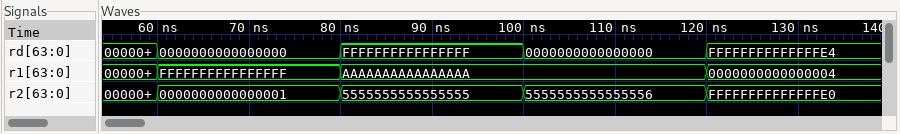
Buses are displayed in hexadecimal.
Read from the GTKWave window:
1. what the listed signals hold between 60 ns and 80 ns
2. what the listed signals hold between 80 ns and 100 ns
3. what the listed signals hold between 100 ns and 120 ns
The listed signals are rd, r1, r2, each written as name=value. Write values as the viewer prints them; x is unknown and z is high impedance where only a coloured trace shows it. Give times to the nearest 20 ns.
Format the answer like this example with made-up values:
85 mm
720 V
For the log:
rd=0000000000000000, r1=FFFFFFFFFFFFFFFF, r2=0000000000000001
rd=FFFFFFFFFFFFFFFF, r1=AAAAAAAAAAAAAAAA, r2=5555555555555555
rd=0000000000000000, r1=AAAAAAAAAAAAAAAA, r2=5555555555555556
